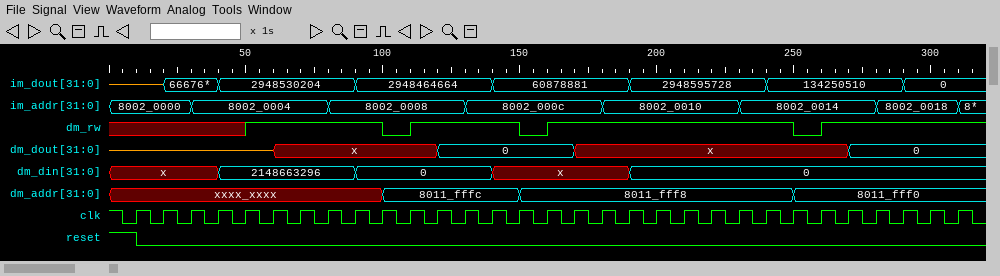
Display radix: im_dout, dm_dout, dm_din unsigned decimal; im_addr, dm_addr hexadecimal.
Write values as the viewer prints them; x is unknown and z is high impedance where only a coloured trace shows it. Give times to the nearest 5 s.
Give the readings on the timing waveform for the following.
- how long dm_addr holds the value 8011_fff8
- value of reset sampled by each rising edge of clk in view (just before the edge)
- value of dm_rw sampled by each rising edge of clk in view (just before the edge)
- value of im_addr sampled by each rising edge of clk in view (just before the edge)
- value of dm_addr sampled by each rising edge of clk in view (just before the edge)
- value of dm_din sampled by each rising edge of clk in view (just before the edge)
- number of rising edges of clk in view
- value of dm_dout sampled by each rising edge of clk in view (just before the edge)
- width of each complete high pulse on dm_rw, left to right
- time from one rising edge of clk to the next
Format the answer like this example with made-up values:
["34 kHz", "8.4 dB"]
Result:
["100 s", "1 0 0 0 0 0 0 0 0 0 0 0 0 0 0 0 0 0 0 0 0 0 0 0 0 0 0 0 0 0 0", "x x x x x 1 1 1 1 1 0 1 1 1 1 0 1 1 1 1 1 1 1 1 1 0 1 1 1 1 1", "8002_0000, 8002_0000, 8002_0000, 8002_0004, 8002_0004, 8002_0004, 8002_0004, 8002_0004, 8002_0008, 8002_0008, 8002_0008, 8002_0008, 8002_0008, 8002_000c, 8002_000c, 8002_000c, 8002_000c, 8002_000c, 8002_0010, 8002_0010, 8002_0010, 8002_0010, 8002_0010, 8002_0014, 8002_0014, 8002_0014, 8002_0014, 8002_0014, 8002_0018, 8002_0018, 8002_0018", "xxxx_xxxx, xxxx_xxxx, xxxx_xxxx, xxxx_xxxx, xxxx_xxxx, xxxx_xxxx, xxxx_xxxx, xxxx_xxxx, xxxx_xxxx, xxxx_xxxx, 8011_fffc, 8011_fffc, 8011_fffc, 8011_fffc, 8011_fffc, 8011_fff8, 8011_fff8, 8011_fff8, 8011_fff8, 8011_fff8, 8011_fff8, 8011_fff8, 8011_fff8, 8011_fff8, 8011_fff8, 8011_fff0, 8011_fff0, 8011_fff0, 8011_fff0, 8011_fff0, 8011_fff0", "x, x, x, x, 2148663296, 2148663296, 2148663296, 2148663296, 2148663296, 0, 0, 0, 0, 0, x, x, x, x, x, 0, 0, 0, 0, 0, 0, 0, 0, 0, 0, 0, 0", "31", "z, z, z, z, z, z, x, x, x, x, x, x, 0, 0, 0, 0, 0, x, x, x, x, x, x, x, x, x, x, 0, 0, 0, 0", "40 s, 90 s", "10 s"]
